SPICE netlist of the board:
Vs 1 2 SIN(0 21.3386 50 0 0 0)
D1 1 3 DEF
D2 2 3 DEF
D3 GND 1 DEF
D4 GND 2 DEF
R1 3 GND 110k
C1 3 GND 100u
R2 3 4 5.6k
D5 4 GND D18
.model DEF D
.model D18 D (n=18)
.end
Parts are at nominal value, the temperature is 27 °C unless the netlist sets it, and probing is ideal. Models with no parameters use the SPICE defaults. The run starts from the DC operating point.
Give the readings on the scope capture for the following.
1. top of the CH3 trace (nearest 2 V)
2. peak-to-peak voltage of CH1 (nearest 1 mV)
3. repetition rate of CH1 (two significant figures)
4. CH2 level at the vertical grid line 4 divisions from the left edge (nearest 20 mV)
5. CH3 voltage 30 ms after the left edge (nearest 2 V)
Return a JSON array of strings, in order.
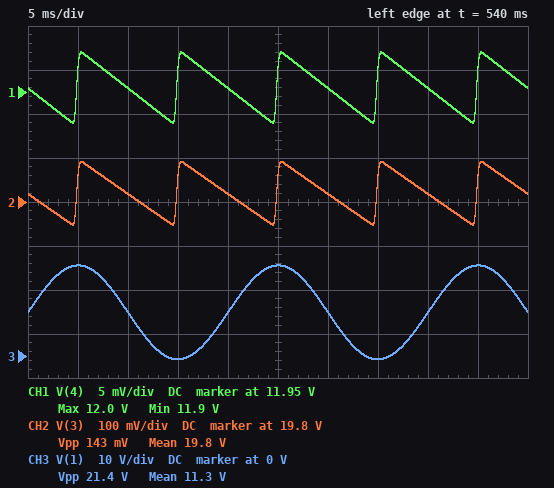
["20 V", "8 mV", "100 Hz", "19.82 V", "10 V"]
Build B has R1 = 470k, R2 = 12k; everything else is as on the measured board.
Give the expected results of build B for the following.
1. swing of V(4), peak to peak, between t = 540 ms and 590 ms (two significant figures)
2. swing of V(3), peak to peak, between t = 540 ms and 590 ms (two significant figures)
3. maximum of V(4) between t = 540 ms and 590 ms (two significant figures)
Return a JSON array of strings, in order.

["3.5 mV", "66 mV", "12 V"]
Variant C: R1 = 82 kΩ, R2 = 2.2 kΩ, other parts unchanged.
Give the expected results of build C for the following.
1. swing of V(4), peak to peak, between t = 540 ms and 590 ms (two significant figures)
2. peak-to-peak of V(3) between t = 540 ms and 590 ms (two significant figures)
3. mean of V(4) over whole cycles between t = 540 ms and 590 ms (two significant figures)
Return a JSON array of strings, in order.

["19 mV", "320 mV", "12 V"]
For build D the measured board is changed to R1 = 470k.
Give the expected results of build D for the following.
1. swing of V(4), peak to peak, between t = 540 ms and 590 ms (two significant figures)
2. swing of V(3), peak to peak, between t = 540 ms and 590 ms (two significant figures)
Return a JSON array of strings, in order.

["7.3 mV", "130 mV"]
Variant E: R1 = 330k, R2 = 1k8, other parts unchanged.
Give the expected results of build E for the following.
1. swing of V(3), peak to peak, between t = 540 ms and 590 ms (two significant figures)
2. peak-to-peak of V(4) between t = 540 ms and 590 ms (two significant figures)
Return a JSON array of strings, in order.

["370 mV", "22 mV"]
